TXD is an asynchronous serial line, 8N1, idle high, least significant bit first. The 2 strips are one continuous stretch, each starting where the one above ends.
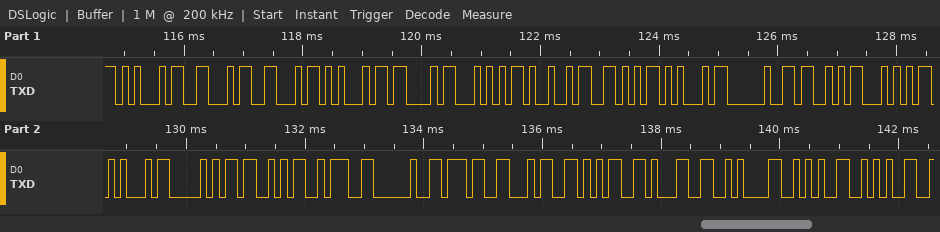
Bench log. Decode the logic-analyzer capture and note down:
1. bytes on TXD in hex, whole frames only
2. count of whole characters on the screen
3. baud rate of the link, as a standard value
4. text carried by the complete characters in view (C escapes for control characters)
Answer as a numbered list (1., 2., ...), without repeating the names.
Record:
1. 0x45 0x46 0x46 0x45 0x43 0x54 0x49 0x56 0x45 0x20 0x53 0x54 0x45 0x50 0x53 0x3A 0x20 0x37 0x34 0x35 0x31 0x0A 0x2A 0x2A
2. 24
3. 9600 baud
4. "EFFECTIVE STEPS: 7451\n**"
